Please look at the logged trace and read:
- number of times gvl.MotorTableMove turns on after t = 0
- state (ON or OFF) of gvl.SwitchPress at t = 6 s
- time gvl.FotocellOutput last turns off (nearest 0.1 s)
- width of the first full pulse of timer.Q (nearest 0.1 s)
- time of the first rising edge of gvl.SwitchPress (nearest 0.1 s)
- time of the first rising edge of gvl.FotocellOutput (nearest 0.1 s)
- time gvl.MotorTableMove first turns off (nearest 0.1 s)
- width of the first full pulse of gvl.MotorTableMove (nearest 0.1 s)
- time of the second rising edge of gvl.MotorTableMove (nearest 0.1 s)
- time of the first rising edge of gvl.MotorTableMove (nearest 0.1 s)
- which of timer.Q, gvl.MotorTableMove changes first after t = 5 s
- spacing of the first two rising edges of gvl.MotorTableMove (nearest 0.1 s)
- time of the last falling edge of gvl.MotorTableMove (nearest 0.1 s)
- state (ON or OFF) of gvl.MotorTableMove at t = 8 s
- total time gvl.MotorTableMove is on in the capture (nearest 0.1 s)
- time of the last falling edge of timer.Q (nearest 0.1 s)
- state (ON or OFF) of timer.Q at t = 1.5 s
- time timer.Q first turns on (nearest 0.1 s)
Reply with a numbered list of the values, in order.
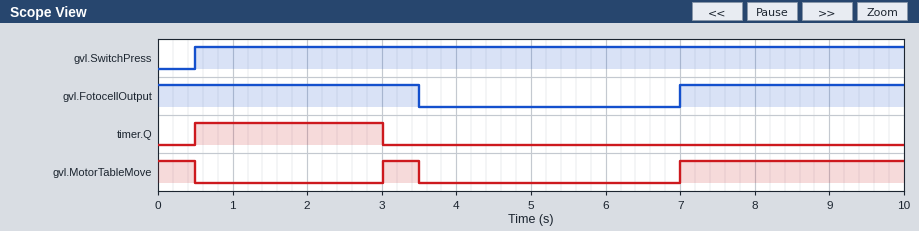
1. 2
2. ON
3. 3.5 s
4. 2.5 s
5. 0.5 s
6. 7.0 s
7. 0.5 s
8. 0.5 s
9. 7.0 s
10. 3.0 s
11. gvl.MotorTableMove
12. 4.0 s
13. 3.5 s
14. ON
15. 4.0 s
16. 3.0 s
17. ON
18. 0.5 s
